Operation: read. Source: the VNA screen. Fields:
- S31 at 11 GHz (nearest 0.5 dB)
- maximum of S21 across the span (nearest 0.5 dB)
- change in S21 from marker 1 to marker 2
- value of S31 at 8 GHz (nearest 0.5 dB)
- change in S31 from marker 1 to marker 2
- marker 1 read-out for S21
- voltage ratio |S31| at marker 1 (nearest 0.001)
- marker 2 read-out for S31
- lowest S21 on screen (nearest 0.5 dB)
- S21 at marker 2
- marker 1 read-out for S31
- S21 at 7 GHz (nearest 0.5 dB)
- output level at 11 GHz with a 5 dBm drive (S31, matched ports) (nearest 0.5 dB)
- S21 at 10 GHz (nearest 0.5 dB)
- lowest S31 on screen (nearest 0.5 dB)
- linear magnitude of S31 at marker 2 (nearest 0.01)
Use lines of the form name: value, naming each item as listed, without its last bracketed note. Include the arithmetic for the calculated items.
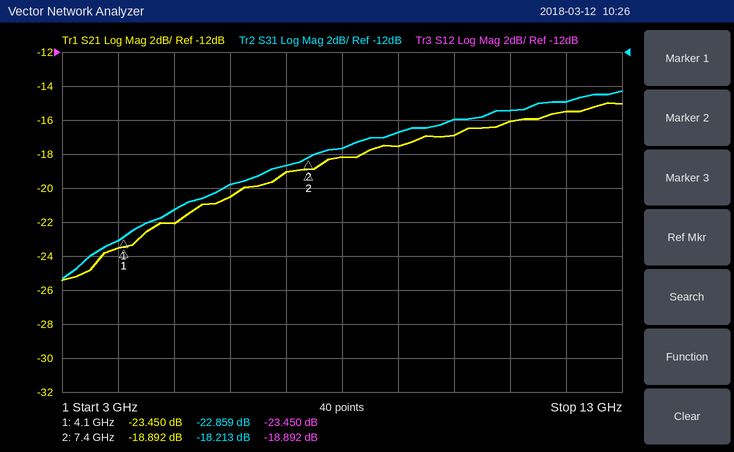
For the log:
S31 at 11 GHz: -15.5 dB
maximum of S21 across the span: -15.0 dB
change in S21 from marker 1 to marker 2: -18.892 − (-23.45) = 4.558 dB
value of S31 at 8 GHz: -17.5 dB
change in S31 from marker 1 to marker 2: -18.213 − (-22.859) = 4.646 dB
marker 1 read-out for S21: -23.450 dB
voltage ratio |S31| at marker 1: 10^(-22.859/20) ≈ 0.072
marker 2 read-out for S31: -18.213 dB
lowest S21 on screen: -25.5 dB
S21 at marker 2: -18.892 dB
marker 1 read-out for S31: -22.859 dB
S21 at 7 GHz: -19.0 dB
output level at 11 GHz with a 5 dBm drive (S31, matched ports): 5 dBm + (-15.5 dB) = -10.5 dBm
S21 at 10 GHz: -17.0 dB
lowest S31 on screen: -25.5 dB
linear magnitude of S31 at marker 2: 10^(-18.213/20) ≈ 0.12
